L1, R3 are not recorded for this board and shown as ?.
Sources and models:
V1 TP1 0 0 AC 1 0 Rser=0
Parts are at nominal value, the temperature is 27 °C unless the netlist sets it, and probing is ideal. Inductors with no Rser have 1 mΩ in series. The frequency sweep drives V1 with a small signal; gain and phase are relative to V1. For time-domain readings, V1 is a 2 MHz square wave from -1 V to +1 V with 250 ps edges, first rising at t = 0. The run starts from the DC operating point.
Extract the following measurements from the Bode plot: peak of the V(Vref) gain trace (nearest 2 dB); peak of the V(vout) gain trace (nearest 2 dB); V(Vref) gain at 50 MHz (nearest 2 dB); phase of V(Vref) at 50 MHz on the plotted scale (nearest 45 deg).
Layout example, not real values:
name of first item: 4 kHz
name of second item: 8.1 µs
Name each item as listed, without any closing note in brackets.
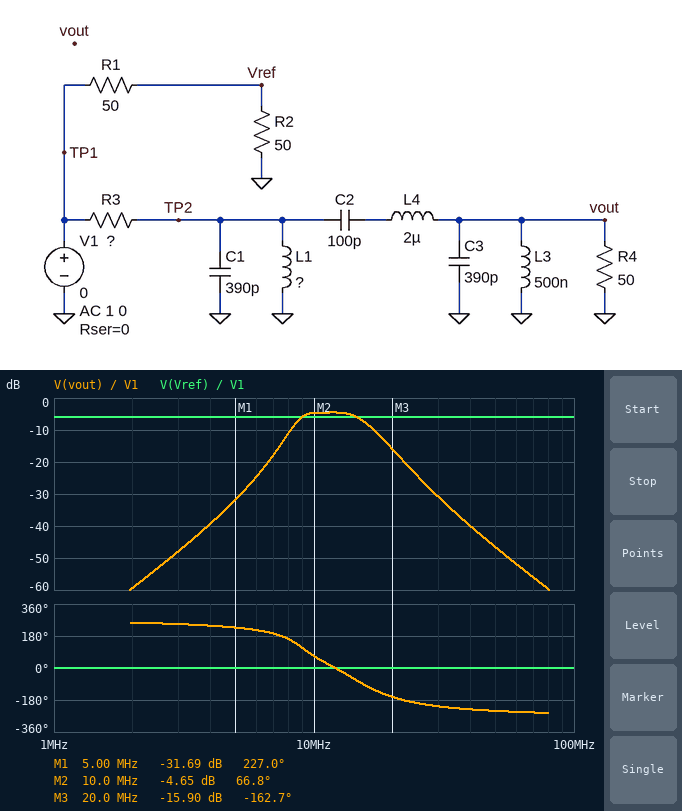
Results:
peak of the V(Vref) gain trace: -6 dB
peak of the V(vout) gain trace: -4 dB
V(Vref) gain at 50 MHz: -6 dB
phase of V(Vref) at 50 MHz on the plotted scale: 0 deg
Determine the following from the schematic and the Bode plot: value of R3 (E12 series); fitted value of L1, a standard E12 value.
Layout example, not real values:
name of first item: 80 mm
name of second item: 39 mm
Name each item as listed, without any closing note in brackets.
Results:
value of R3: 27 Ω
fitted value of L1, a standard E12 value: 270 nH
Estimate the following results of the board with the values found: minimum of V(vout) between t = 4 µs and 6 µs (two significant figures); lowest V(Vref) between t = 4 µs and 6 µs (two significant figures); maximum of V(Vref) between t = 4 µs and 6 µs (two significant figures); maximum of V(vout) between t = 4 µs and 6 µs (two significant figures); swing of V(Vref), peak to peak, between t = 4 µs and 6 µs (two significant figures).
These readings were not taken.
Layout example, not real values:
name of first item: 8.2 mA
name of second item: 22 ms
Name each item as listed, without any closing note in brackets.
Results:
minimum of V(vout) between t = 4 µs and 6 µs: -290 mV
lowest V(Vref) between t = 4 µs and 6 µs: -500 mV
maximum of V(Vref) between t = 4 µs and 6 µs: 500 mV
maximum of V(vout) between t = 4 µs and 6 µs: 290 mV
swing of V(Vref), peak to peak, between t = 4 µs and 6 µs: 1.0 V
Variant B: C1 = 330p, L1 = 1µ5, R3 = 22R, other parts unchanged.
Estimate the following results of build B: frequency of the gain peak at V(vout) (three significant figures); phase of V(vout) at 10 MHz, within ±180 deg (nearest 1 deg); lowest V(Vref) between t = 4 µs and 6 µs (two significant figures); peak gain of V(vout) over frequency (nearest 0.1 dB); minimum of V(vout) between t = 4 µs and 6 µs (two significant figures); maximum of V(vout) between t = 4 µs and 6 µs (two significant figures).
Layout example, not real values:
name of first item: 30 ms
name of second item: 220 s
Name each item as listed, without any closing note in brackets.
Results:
frequency of the gain peak at V(vout): 11.1 MHz
phase of V(vout) at 10 MHz, within ±180 deg: 26 deg
lowest V(Vref) between t = 4 µs and 6 µs: -500 mV
peak gain of V(vout) over frequency: -3.3 dB
minimum of V(vout) between t = 4 µs and 6 µs: -370 mV
maximum of V(vout) between t = 4 µs and 6 µs: 370 mV
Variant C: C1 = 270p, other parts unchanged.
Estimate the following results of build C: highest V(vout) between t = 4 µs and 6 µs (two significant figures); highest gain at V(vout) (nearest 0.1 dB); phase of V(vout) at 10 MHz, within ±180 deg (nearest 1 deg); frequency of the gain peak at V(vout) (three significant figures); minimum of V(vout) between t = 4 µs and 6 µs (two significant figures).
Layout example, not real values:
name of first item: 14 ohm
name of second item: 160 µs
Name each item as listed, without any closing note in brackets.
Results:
highest V(vout) between t = 4 µs and 6 µs: 270 mV
highest gain at V(vout): -5.1 dB
phase of V(vout) at 10 MHz, within ±180 deg: 73 deg
frequency of the gain peak at V(vout): 11.6 MHz
minimum of V(vout) between t = 4 µs and 6 µs: -270 mV
